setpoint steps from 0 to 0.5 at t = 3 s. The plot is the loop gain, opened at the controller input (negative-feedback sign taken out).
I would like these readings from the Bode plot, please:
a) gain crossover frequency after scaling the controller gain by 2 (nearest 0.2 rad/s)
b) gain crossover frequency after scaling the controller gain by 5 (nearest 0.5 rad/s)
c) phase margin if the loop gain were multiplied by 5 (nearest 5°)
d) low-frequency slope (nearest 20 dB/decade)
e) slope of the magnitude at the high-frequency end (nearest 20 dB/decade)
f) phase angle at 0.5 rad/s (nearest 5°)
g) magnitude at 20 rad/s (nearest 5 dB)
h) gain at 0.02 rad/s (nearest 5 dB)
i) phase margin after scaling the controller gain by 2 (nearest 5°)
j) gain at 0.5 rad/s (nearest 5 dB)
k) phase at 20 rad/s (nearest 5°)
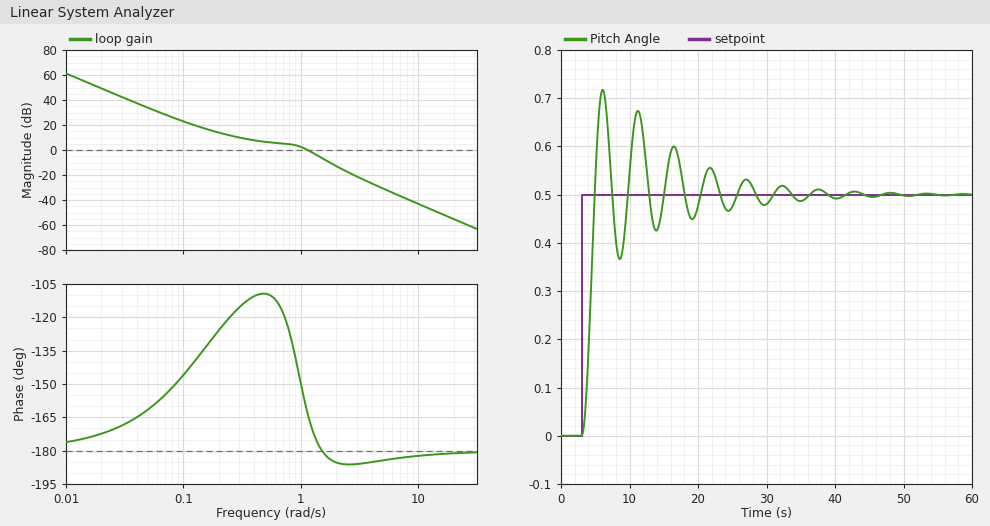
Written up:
1.4 rad/s
2.0 rad/s
-5°
-40 dB/decade
-40 dB/decade
-110°
-55 dB
50 dB
0°
5 dB
-180°
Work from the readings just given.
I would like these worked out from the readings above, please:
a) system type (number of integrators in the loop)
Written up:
2
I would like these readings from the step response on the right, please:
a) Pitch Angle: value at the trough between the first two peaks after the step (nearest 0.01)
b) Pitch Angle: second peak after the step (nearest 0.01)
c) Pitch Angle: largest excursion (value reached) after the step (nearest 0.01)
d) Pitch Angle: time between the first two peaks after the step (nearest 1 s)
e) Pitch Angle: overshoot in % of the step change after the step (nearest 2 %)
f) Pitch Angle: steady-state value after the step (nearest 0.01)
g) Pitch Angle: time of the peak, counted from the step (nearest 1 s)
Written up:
0.37
0.67
0.72
5 s
44 %
0.50
3 s
